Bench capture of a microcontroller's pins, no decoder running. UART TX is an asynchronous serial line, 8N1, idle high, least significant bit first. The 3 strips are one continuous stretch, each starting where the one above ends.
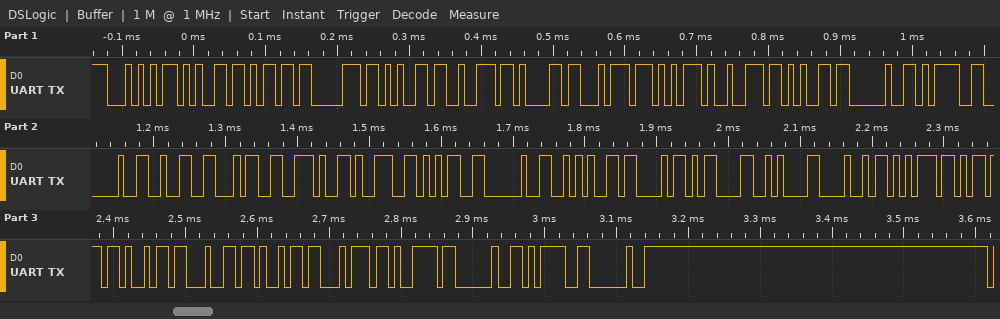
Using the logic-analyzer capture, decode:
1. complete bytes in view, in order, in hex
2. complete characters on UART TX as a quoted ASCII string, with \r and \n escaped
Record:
54 65 6D 70 65 72 61 74 75 72 65 20 3D 20 32 34 2E 39 35 20 2A 43 0D 0A 48 75 6D 69 64 69 74 79 20 3D 20
"Temperature = 24.95 *C\r\nHumidity = "
